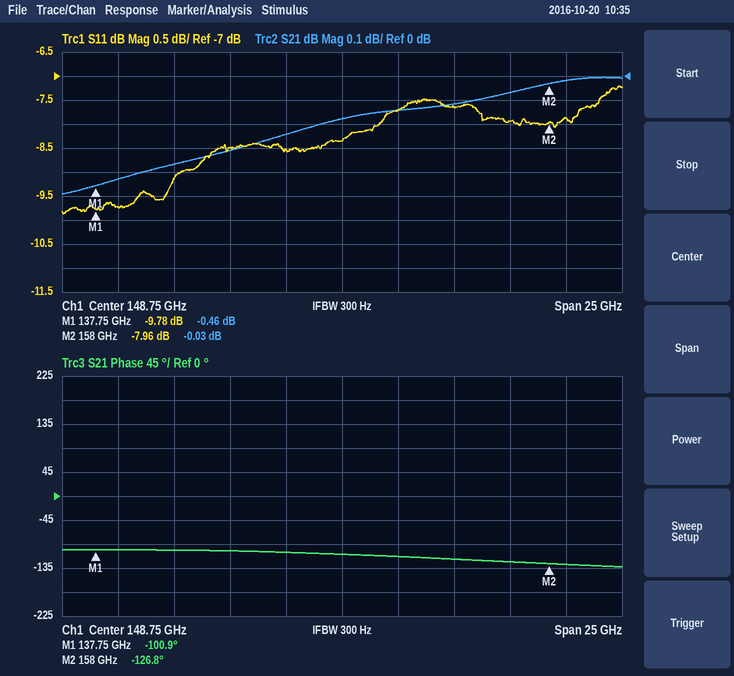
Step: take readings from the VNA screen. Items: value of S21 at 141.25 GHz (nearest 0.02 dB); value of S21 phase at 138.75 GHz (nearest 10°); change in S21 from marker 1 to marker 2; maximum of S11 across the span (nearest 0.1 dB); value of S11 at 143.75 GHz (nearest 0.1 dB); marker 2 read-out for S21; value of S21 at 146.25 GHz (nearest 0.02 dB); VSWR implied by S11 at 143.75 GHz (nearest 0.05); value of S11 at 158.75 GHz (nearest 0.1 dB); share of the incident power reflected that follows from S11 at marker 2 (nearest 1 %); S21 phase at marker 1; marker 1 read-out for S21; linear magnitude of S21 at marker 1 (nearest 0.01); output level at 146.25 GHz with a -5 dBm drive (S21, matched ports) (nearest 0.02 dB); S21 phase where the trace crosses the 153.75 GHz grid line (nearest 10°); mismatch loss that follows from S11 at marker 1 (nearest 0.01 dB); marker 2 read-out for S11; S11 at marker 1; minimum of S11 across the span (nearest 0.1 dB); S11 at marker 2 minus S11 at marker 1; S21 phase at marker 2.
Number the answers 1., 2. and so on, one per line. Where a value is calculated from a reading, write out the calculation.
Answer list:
1. -0.36 dB
2. -100°
3. -0.03 − (-0.46) = 0.43 dB
4. -7.2 dB
5. -8.5 dB
6. -0.03 dB
7. -0.24 dB
8. |Γ| = 10^(-8.5/20) = 0.3758; VSWR = (1 + 0.3758)/(1 − 0.3758) ≈ 2.20
9. -7.9 dB
10. 10^(-7.96/10) ≈ 16 %
11. -100.9°
12. -0.46 dB
13. 10^(-0.46/20) ≈ 0.95
14. -5 dBm + (-0.24 dB) = -5.24 dBm
15. -120°
16. −10 log10(1 − 10^(-9.78/10)) ≈ 0.48 dB
17. -7.96 dB
18. -9.78 dB
19. -9.9 dB
20. -7.96 − (-9.78) = 1.82 dB
21. -126.8°
